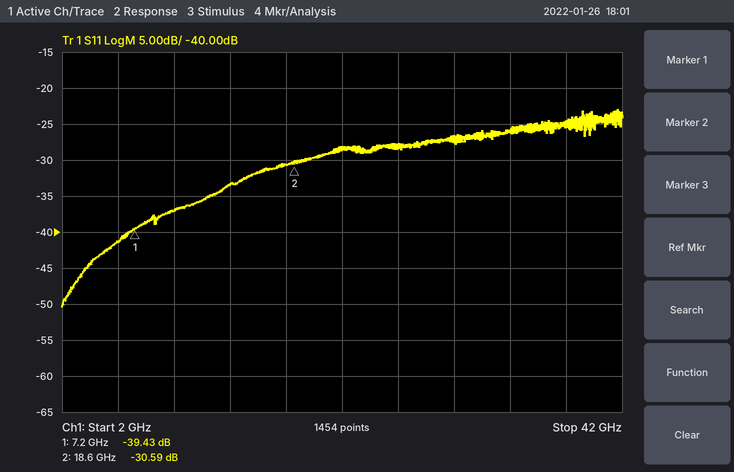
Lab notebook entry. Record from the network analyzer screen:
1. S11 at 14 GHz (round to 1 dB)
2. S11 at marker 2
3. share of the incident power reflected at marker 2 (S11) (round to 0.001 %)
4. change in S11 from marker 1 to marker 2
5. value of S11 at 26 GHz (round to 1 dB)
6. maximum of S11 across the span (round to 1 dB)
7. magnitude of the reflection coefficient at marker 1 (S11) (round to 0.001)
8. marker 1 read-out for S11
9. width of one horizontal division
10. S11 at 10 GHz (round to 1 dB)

-33 dB
-30.59 dB
0.087 %
8.84 dB
-28 dB
-23 dB
0.011
-39.43 dB
4 GHz
-37 dB
